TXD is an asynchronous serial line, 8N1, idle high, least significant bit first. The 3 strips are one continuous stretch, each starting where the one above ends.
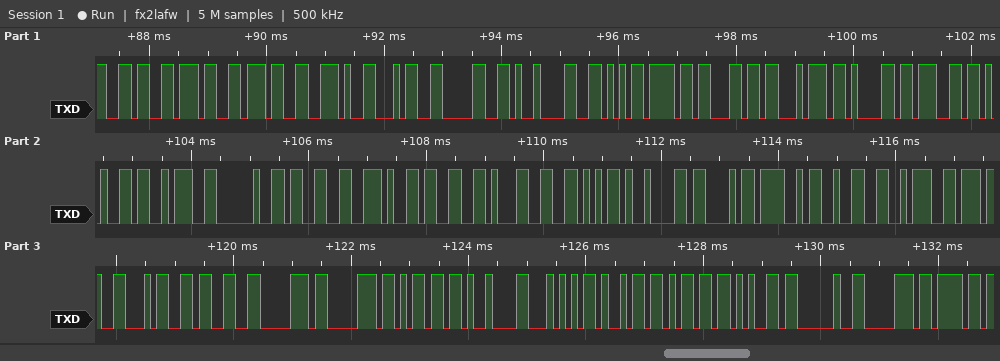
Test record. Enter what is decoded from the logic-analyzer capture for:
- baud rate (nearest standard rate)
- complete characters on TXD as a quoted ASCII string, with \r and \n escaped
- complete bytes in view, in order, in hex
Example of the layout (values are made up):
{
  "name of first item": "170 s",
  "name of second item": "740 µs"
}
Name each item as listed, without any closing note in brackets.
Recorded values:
{
  "baud rate": "9600 baud",
  "complete characters on TXD as a quoted ASCII string, with \\r and \\n escaped": "\"677.40\\tVoltage: 3.31V\\tCO2:743ppm\\tTime po\"",
  "complete bytes in view, in order, in hex": "36 37 37 2E 34 30 09 56 6F 6C 74 61 67 65 3A 20 33 2E 33 31 56 09 43 4F 32 3A 37 34 33 70 70 6D 09 54 69 6D 65 20 70 6F"
}
